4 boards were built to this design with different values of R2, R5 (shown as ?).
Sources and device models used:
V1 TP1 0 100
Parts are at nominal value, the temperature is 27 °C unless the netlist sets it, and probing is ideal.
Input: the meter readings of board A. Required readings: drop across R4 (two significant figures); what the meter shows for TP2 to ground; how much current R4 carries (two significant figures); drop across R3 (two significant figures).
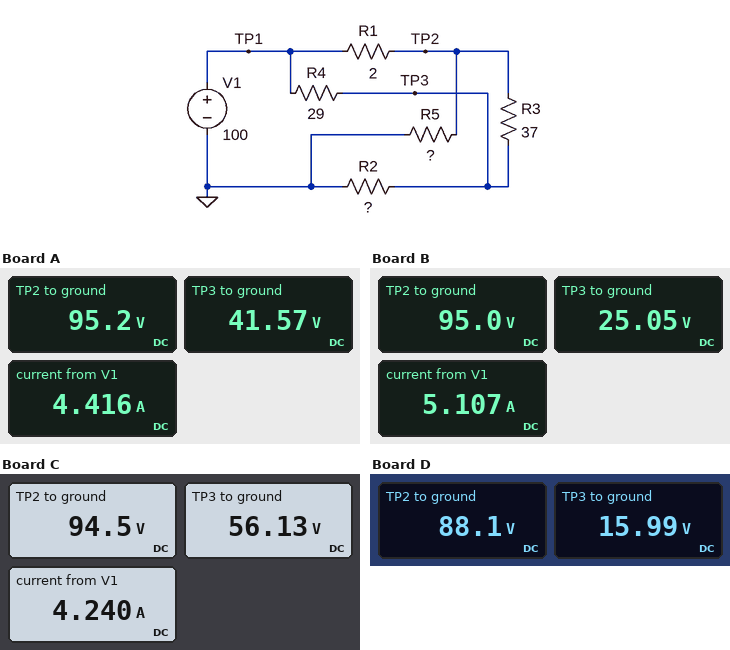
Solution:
58 V
95.2 V
2.0 A
54 V
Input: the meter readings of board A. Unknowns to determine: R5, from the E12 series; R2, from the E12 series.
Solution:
100 Ω
12 Ω
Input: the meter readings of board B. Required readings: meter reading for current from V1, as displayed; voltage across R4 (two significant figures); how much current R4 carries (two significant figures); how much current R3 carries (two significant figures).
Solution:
5.107 A
75 V
2.6 A
1.9 A
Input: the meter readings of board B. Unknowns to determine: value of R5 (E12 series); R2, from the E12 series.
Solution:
150 Ω
5.6 Ω
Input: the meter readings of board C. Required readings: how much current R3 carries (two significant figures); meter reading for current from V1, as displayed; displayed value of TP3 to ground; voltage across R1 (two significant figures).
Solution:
1.0 A
4.240 A
56.13 V
5.5 V
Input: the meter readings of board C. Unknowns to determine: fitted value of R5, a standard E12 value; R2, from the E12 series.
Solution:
56 Ω
22 Ω
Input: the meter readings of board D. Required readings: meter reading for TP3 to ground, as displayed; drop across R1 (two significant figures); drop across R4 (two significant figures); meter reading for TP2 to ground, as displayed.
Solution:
15.99 V
12 V
84 V
88.1 V
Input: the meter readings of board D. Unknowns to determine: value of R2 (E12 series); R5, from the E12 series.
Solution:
3.3 Ω
22 Ω
